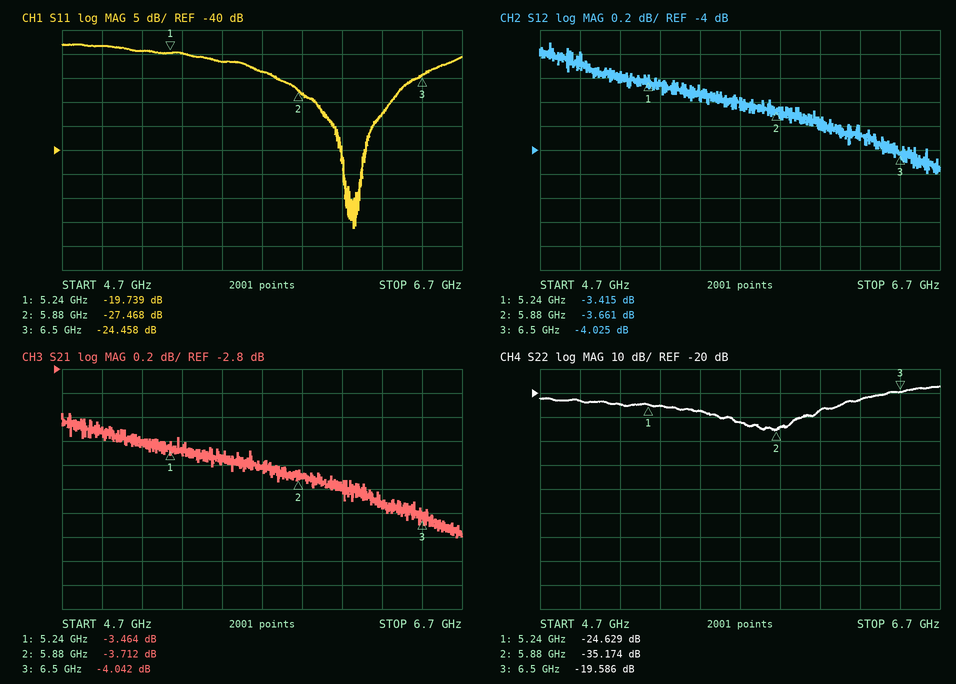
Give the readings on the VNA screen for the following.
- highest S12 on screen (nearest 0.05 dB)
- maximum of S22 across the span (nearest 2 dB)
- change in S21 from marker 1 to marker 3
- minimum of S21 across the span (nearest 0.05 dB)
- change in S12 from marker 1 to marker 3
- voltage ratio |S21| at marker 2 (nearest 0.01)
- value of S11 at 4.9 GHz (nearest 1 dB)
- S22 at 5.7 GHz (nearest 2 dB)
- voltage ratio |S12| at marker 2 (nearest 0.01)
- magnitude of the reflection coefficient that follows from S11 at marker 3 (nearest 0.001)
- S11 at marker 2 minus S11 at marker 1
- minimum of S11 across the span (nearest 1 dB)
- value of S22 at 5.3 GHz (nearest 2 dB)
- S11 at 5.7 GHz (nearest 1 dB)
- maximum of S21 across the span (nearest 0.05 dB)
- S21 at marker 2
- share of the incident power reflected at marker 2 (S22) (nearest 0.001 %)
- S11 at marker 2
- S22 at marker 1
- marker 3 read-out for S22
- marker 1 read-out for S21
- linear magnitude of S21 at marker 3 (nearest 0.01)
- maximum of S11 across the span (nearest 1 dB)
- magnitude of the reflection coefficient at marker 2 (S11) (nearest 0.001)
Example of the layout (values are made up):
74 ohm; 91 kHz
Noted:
-3.10 dB; -18 dB; -0.578 dB; -4.20 dB; -0.610 dB; 0.65; -18 dB; -32 dB; 0.66; 0.060; -7.729 dB; -56 dB; -26 dB; -24 dB; -3.15 dB; -3.712 dB; 0.030 %; -27.468 dB; -24.629 dB; -19.586 dB; -3.464 dB; 0.63; -18 dB; 0.042
